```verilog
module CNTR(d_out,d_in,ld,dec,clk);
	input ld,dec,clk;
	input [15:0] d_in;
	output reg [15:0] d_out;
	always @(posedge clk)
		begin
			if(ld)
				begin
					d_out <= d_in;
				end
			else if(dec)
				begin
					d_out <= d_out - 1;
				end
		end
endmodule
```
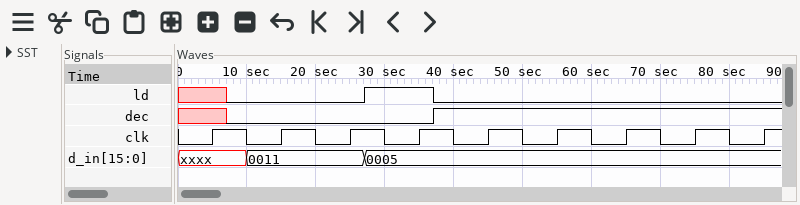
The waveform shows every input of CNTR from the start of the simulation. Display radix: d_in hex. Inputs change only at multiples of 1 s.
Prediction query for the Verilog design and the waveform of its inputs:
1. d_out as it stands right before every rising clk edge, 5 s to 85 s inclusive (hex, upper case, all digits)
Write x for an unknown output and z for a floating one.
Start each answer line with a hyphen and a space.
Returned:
- x, x, x, x, 0005, 0004, 0003, 0002, 0001
